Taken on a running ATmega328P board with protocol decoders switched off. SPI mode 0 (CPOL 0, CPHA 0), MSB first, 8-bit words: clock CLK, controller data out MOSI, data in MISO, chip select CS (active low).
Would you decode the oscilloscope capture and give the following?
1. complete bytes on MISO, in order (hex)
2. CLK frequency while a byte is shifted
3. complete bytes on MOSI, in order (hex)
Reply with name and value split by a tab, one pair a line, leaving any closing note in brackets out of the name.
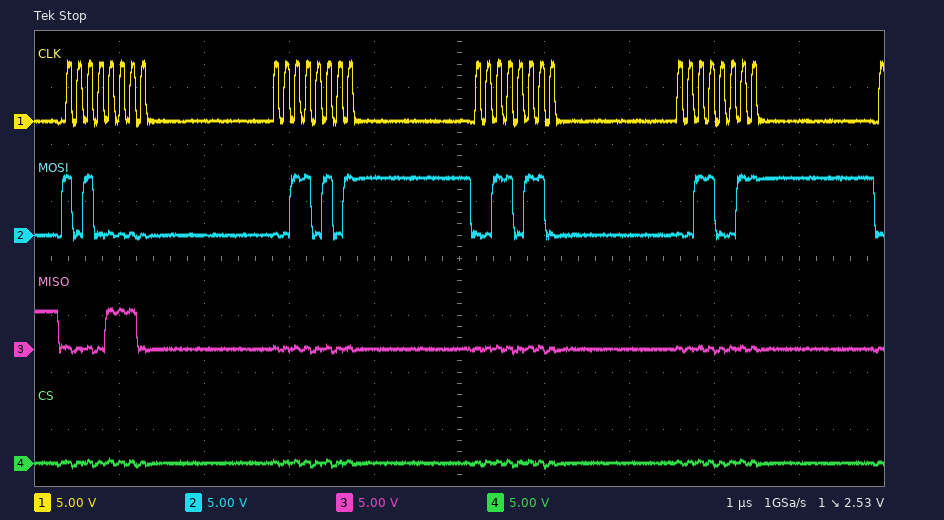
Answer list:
complete bytes on MISO, in order	0x0E 0x00 0x00 0x00
CLK frequency while a byte is shifted	8 MHz
complete bytes on MOSI, in order	0xA0 0x35 0x36 0x33
